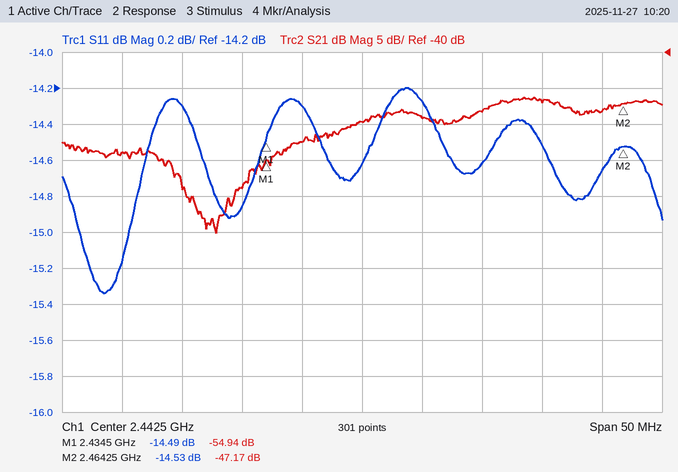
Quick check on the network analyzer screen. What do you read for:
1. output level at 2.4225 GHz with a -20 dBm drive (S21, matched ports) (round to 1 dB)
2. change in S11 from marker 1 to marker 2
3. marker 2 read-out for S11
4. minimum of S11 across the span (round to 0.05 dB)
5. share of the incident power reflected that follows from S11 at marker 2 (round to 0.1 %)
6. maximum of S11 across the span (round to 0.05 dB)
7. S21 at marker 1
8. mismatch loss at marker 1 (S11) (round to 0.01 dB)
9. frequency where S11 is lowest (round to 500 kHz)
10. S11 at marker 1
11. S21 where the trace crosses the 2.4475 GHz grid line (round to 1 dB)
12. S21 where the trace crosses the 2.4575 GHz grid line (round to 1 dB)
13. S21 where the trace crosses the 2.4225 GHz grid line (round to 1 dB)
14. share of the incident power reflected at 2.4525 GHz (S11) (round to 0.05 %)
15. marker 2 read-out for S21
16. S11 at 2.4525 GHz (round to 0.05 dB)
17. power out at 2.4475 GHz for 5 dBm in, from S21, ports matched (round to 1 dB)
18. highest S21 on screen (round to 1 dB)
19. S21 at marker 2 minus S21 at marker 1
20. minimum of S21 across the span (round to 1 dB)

-74 dBm
-0.04 dB
-14.53 dB
-15.35 dB
3.5 %
-14.20 dB
-54.94 dB
0.16 dB
2.4210 GHz
-14.49 dB
-49 dB
-47 dB
-54 dB
3.45 %
-47.17 dB
-14.60 dB
-44 dBm
-46 dB
7.77 dB
-65 dB
